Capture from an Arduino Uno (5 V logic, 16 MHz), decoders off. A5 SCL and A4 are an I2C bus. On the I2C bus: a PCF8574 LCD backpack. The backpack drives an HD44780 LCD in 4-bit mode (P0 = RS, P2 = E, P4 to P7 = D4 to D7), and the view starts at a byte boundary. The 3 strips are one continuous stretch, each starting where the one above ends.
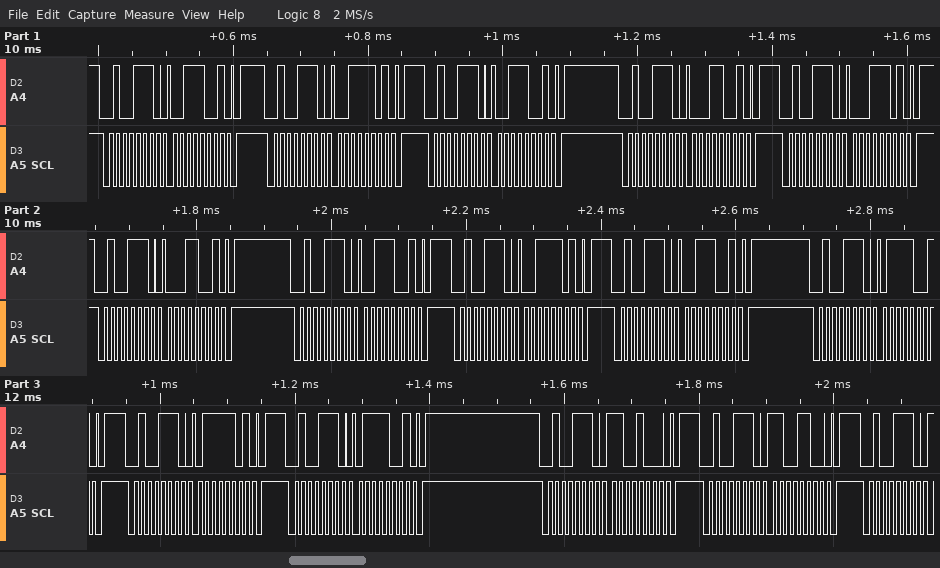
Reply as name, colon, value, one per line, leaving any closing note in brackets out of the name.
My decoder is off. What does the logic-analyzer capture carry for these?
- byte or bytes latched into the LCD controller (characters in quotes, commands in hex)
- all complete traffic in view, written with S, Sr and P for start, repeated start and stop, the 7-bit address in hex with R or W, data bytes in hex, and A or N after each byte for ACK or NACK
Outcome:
byte or bytes latched into the LCD controller: '1' '7'
all complete traffic in view, written with S, Sr and P for start, repeated start and stop, the 7-bit address in hex with R or W, data bytes in hex, and A or N after each byte for ACK or NACK: S 27W A 39 A P S 27W A 3D A P S 27W A 39 A P S 27W A 19 A P S 27W A 1D A P S 27W A 19 A P S 27W A 39 A P S 27W A 3D A P S 27W A 39 A P S 27W A 79 A P S 27W A 7D A P S 27W A 79 A P S 27W A C8 A P S 27W A CC A P S 27W A
